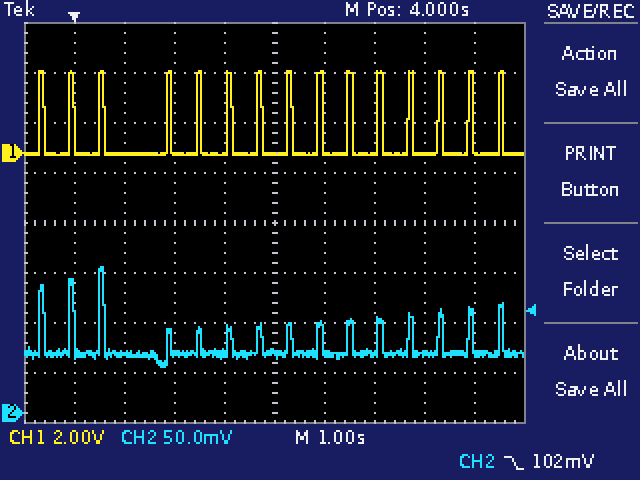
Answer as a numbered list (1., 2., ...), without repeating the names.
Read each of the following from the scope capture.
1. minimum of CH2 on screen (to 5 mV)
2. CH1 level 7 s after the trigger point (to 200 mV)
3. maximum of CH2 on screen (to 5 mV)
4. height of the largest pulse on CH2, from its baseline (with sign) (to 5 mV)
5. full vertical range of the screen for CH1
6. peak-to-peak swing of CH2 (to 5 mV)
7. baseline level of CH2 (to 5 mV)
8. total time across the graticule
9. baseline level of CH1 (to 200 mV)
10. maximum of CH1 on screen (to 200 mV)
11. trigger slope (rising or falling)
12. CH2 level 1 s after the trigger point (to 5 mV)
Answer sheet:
1. 45 mV
2. 0.0 V
3. 145 mV
4. +85 mV
5. 16 V
6. 100 mV
7. 60 mV
8. 10 s
9. 0.0 V
10. 3.2 V
11. falling
12. 60 mV
